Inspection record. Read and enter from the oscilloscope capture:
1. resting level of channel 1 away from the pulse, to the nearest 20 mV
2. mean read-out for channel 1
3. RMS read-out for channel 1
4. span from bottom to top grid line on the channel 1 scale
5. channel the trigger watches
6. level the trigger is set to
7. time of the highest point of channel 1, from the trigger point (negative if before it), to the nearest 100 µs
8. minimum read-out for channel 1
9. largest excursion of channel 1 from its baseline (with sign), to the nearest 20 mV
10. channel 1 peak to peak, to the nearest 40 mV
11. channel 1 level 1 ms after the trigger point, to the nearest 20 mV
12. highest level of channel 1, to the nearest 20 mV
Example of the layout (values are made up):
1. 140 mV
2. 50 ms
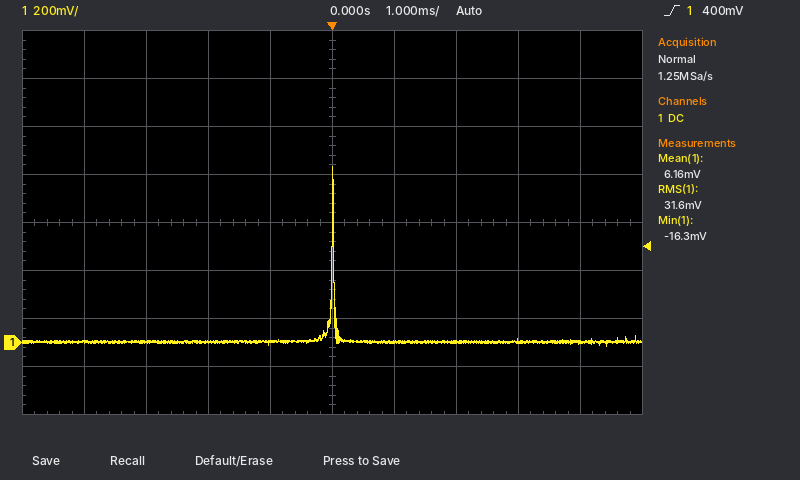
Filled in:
1. 0 mV
2. 6.16 mV
3. 31.6 mV
4. 1.6 V
5. channel 1
6. 400 mV
7. 0.0 ms
8. -16.3 mV
9. +740 mV
10. 760 mV
11. 0 mV
12. 740 mV
